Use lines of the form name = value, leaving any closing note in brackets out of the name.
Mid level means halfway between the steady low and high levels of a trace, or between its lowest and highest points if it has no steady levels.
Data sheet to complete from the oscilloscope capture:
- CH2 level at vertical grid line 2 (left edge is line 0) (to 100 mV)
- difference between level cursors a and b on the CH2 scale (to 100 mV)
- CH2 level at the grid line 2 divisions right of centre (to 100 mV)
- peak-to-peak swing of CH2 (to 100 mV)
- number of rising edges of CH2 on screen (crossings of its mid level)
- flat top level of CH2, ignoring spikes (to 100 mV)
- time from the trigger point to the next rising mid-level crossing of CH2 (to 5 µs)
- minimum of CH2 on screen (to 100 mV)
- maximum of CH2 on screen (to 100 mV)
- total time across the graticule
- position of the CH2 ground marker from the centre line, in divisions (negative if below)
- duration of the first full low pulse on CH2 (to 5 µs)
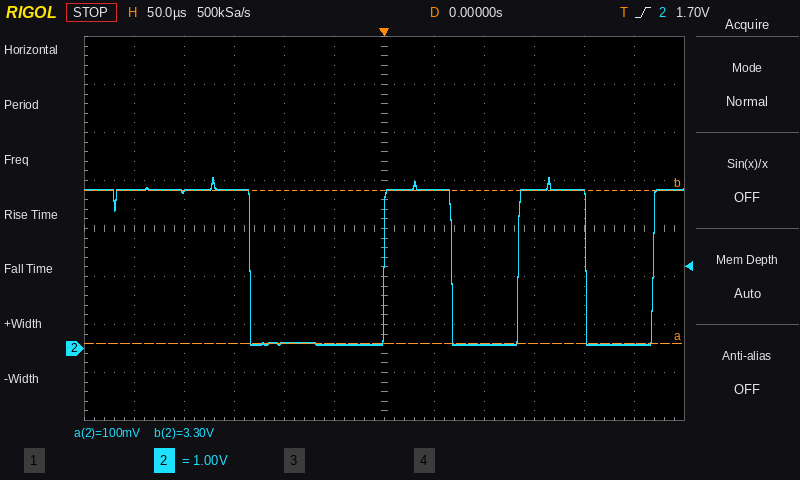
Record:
CH2 level at vertical grid line 2 (left edge is line 0) = 3.3 V
difference between level cursors a and b on the CH2 scale = 3.2 V
CH2 level at the grid line 2 divisions right of centre = 100 mV
peak-to-peak swing of CH2 = 3.5 V
number of rising edges of CH2 on screen = 3
flat top level of CH2, ignoring spikes = 3.3 V
time from the trigger point to the next rising mid-level crossing of CH2 = 135 µs
minimum of CH2 on screen = 100 mV
maximum of CH2 on screen = 3.6 V
total time across the graticule = 600 µs
position of the CH2 ground marker from the centre line, in divisions = -2.5 div
duration of the first full low pulse on CH2 = 135 µs
